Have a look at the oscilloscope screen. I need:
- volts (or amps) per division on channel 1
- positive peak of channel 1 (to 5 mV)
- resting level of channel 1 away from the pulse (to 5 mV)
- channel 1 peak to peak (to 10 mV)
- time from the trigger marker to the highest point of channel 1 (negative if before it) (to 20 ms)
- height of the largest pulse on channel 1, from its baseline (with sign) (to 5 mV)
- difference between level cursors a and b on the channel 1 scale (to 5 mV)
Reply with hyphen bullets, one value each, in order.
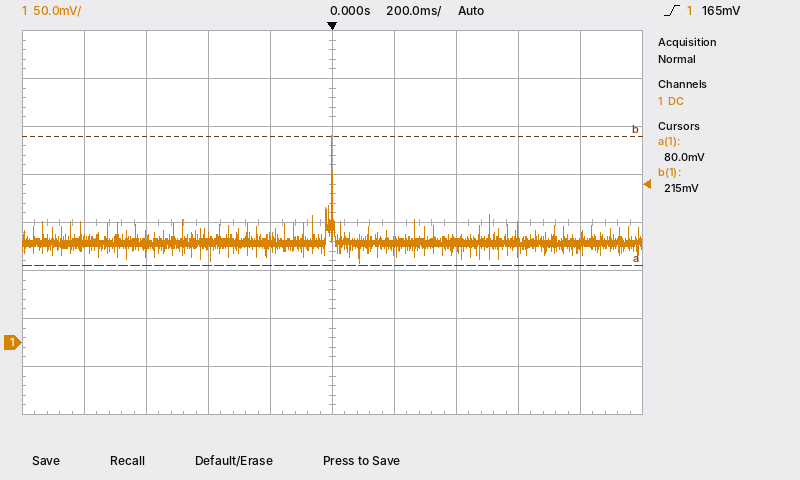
- 50 mV
- 215 mV
- 105 mV
- 130 mV
- 0 ms
- +110 mV
- 135 mV
